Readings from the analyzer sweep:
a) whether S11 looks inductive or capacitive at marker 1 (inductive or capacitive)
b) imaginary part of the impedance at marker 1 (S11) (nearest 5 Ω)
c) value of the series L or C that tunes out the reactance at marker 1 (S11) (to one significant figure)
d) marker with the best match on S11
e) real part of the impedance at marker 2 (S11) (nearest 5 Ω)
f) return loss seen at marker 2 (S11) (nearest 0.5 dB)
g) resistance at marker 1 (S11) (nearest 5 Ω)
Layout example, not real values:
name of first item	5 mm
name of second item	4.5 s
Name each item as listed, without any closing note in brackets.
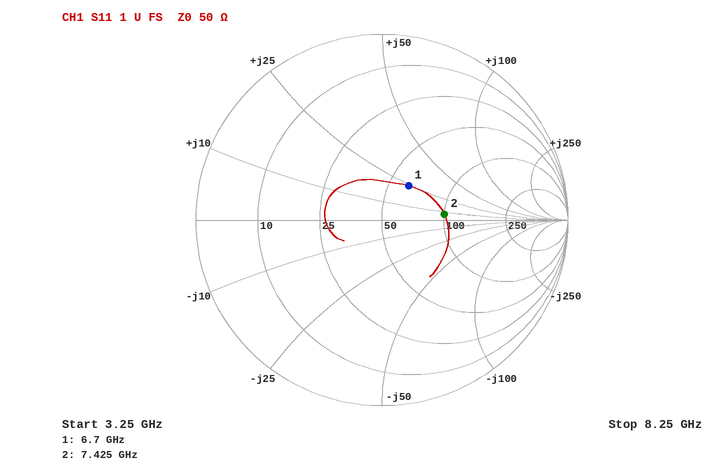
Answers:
whether S11 looks inductive or capacitive at marker 1	inductive
imaginary part of the impedance at marker 1 (S11)	+25 Ω
value of the series L or C that tunes out the reactance at marker 1 (S11)	1.0 pF
marker with the best match on S11	marker 1
real part of the impedance at marker 2 (S11)	100 Ω
return loss seen at marker 2 (S11)	9.5 dB
resistance at marker 1 (S11)	60 Ω
